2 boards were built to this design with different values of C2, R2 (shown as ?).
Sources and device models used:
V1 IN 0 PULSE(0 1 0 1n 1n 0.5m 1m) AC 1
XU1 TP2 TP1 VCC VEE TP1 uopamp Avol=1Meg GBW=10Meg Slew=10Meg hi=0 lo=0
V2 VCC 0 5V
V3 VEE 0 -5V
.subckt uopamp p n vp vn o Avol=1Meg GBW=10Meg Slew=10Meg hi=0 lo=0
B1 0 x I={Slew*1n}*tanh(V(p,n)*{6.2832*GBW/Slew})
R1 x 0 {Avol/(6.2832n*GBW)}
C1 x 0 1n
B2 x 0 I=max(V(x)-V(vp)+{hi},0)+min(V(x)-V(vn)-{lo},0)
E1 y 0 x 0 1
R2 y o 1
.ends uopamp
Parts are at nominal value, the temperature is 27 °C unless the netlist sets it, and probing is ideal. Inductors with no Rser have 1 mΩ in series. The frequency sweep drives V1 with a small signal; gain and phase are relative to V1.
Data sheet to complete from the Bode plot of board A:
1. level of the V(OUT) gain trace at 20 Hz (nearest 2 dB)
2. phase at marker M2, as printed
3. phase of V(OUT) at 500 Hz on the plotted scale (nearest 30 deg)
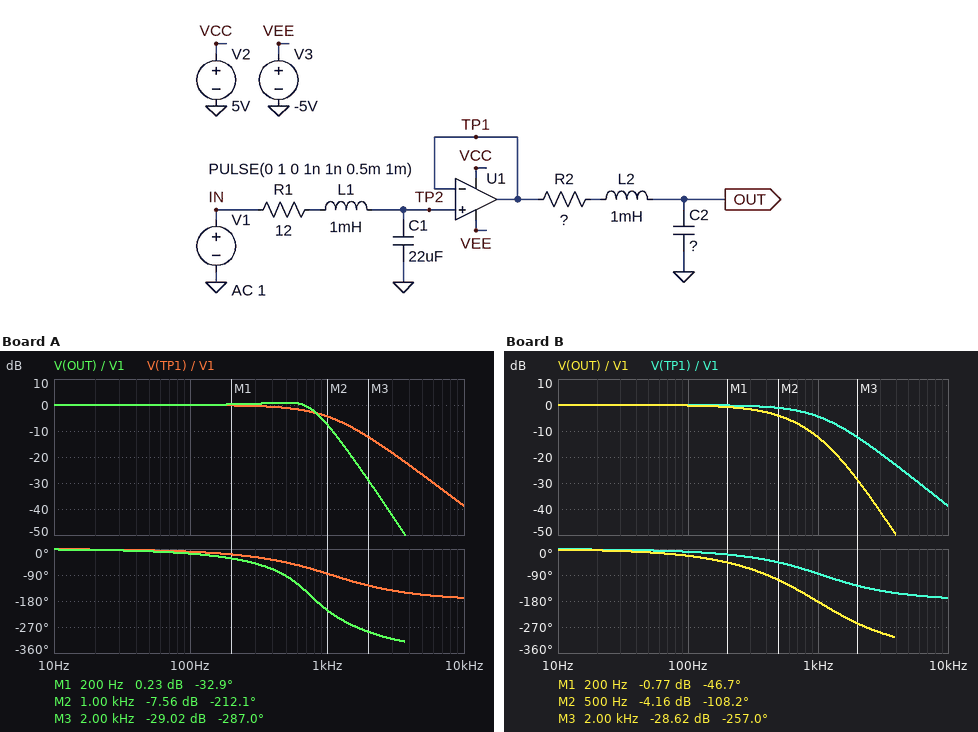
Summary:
0 dB
-212.1 deg
-90 deg
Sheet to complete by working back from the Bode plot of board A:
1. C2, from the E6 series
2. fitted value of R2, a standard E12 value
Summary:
47 µF
3.9 Ω
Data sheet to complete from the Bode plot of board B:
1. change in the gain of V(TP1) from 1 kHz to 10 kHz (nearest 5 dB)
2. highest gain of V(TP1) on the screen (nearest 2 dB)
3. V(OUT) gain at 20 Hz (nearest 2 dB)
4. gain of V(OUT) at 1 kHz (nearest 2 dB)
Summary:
-35 dB
0 dB
0 dB
-12 dB
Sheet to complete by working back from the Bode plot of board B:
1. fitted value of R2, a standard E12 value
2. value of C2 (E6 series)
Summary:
12 Ω
33 µF
